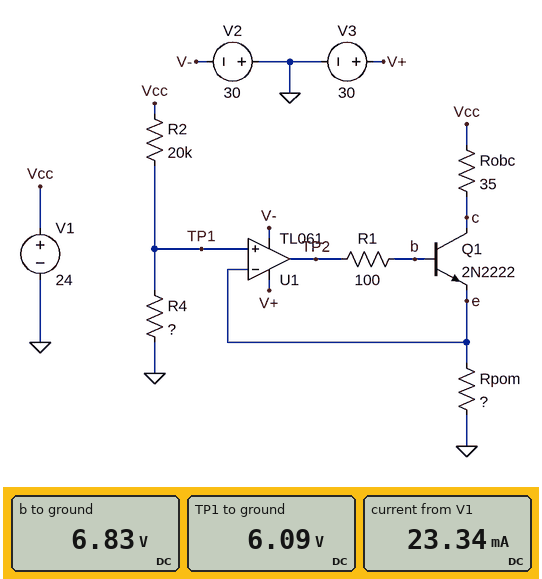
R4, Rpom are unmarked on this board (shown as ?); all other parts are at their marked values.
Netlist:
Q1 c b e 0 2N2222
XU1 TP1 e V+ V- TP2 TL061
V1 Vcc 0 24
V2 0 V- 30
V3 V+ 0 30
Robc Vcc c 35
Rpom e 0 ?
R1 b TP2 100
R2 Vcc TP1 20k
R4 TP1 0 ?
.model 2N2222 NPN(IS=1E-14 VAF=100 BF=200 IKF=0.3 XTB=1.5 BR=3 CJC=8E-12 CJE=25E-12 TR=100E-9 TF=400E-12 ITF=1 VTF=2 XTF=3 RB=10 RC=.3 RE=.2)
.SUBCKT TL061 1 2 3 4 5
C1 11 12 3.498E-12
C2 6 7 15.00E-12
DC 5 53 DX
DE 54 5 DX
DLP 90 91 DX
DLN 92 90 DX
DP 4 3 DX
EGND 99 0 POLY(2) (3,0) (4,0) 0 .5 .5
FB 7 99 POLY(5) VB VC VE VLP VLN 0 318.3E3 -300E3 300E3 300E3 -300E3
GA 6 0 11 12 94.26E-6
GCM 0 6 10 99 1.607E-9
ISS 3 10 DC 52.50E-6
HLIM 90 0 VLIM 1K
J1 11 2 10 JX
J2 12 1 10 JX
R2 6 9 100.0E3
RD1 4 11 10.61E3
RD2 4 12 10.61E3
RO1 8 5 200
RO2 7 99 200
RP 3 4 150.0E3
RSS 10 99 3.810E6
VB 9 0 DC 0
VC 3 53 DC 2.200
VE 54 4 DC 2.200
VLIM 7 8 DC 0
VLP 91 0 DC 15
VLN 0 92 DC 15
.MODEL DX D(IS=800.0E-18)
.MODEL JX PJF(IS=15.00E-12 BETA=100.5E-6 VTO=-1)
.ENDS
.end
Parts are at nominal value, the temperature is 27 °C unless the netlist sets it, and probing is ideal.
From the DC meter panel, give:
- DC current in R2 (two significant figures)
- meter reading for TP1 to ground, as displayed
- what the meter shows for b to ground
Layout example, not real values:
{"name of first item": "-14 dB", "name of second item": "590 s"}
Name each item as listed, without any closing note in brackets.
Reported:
{"DC current in R2": "900 µA", "meter reading for TP1 to ground, as displayed": "6.09 V", "what the meter shows for b to ground": "6.83 V"}
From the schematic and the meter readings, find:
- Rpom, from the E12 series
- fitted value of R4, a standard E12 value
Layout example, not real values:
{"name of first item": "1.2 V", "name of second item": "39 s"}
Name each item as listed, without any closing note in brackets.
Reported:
{"Rpom, from the E12 series": "270 Ω", "fitted value of R4, a standard E12 value": "6.8 kΩ"}
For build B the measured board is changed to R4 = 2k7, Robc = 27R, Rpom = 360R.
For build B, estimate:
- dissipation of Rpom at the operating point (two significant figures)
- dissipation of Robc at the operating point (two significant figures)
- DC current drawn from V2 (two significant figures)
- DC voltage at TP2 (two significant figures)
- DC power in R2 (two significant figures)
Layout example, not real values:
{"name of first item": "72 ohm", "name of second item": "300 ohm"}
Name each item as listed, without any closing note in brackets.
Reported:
{"dissipation of Rpom at the operating point": "23 mW", "dissipation of Robc at the operating point": "1.7 mW", "DC current drawn from V2": "450 µA", "DC voltage at TP2": "3.6 V", "DC power in R2": "22 mW"}
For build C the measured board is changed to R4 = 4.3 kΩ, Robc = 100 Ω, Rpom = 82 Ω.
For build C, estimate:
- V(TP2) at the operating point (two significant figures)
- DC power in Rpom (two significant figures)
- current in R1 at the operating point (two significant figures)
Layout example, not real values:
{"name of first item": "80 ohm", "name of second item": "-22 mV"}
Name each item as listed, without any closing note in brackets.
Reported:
{"V(TP2) at the operating point": "5.0 V", "DC power in Rpom": "220 mW", "current in R1 at the operating point": "260 µA"}
